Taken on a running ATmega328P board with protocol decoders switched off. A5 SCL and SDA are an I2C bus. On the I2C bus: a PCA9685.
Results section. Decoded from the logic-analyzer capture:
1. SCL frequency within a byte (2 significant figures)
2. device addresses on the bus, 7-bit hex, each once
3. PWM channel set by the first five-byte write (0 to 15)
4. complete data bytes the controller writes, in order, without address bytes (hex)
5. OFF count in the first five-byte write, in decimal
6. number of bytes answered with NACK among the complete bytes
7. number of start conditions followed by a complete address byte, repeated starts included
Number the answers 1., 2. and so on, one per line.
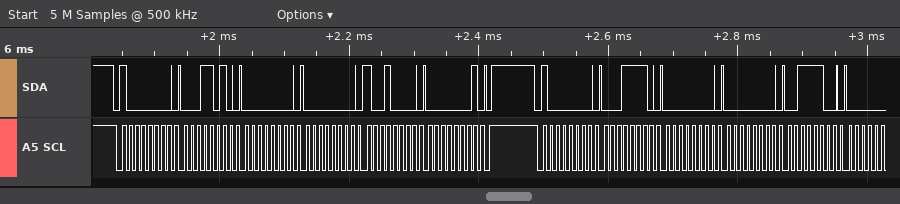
1. 100 kHz
2. 0x40
3. 5
4. 1A 00 00 90 01 1E 00 00 3C
5. 400
6. 0
7. 2
